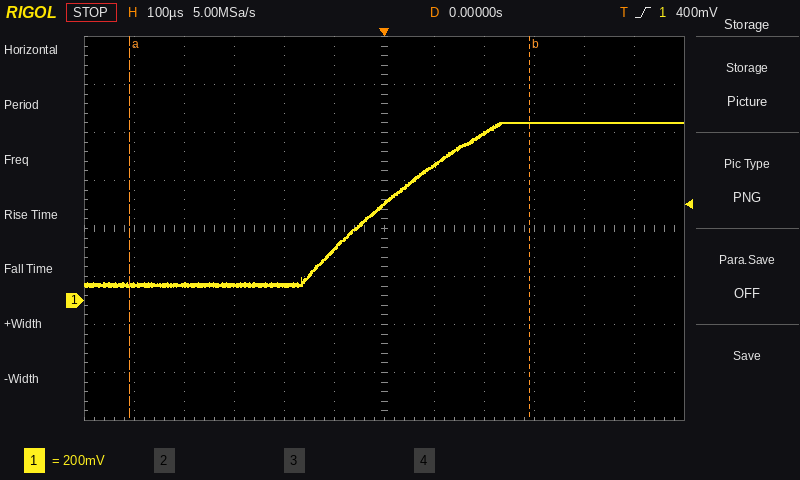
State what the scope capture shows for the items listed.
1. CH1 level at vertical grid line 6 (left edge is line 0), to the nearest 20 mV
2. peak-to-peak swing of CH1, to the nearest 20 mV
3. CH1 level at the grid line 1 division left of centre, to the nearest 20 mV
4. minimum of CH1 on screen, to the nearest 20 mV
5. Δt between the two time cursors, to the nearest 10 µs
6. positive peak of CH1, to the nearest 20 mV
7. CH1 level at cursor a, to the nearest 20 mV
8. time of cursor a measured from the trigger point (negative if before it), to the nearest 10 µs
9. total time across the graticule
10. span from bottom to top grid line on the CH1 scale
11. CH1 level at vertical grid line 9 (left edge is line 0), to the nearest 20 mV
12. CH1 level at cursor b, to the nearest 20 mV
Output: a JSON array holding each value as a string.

["400 mV", "680 mV", "220 mV", "60 mV", "800 µs", "740 mV", "60 mV", "-510 µs", "1.2 ms", "1.6 V", "740 mV", "740 mV"]
